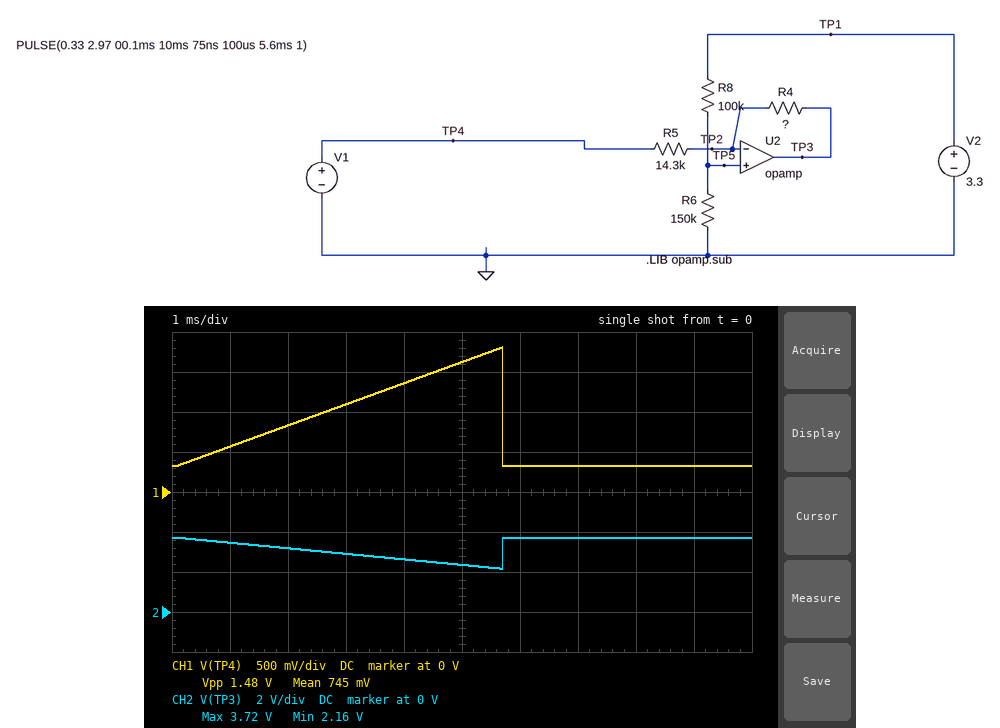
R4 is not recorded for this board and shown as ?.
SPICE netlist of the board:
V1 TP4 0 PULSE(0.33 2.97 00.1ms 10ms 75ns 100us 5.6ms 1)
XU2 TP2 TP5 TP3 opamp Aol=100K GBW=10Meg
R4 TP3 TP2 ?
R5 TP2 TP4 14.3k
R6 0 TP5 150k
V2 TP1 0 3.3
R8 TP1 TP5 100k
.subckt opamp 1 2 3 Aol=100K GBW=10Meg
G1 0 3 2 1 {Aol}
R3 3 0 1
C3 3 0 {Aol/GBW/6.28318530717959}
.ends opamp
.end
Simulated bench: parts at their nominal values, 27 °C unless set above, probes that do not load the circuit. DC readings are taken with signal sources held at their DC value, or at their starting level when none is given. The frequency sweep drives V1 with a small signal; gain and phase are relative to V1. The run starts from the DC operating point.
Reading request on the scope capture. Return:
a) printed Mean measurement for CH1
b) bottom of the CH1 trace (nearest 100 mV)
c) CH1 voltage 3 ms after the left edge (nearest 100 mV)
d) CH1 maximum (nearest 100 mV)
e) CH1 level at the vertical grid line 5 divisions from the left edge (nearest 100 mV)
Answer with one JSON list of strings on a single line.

["745 mV", "300 mV", "1.1 V", "1.8 V", "1.6 V"]
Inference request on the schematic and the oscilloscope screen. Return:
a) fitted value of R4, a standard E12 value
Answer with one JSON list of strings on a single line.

["15 kΩ"]
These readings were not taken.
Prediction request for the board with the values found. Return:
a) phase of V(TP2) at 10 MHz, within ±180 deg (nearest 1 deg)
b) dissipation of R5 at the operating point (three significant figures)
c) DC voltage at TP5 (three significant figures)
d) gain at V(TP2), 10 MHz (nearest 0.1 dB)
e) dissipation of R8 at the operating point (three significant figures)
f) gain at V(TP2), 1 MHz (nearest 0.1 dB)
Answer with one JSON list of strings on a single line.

["26 deg", "190 µW", "1.98 V", "-6.7 dB", "17.4 µW", "-19.8 dB"]
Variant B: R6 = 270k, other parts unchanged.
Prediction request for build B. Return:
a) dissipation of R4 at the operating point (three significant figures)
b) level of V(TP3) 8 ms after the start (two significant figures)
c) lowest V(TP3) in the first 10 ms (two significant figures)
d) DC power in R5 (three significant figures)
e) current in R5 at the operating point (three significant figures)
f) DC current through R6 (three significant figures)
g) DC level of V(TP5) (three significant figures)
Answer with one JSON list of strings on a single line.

["317 µW", "4.6 V", "3.0 V", "302 µW", "145 µA", "8.92 µA", "2.41 V"]
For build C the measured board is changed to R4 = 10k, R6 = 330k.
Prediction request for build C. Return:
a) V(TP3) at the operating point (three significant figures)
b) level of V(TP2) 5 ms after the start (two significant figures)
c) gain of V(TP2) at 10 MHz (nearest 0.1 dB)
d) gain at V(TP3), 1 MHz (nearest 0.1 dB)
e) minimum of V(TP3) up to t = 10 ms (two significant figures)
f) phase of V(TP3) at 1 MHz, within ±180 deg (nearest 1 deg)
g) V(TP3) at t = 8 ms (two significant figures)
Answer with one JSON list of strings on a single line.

["4.07 V", "2.5 V", "-9.0 dB", "-3.2 dB", "3.0 V", "170 deg", "4.1 V"]
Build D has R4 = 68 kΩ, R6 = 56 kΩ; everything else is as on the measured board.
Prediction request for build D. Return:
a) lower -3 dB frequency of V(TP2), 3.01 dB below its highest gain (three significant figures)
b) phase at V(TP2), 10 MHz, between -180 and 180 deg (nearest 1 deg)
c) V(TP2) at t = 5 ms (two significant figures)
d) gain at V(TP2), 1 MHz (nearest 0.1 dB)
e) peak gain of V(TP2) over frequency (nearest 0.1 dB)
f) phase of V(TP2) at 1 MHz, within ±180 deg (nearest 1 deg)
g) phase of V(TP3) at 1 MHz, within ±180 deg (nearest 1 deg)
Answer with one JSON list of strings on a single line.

["1.74 MHz", "10 deg", "1.2 V", "-7.7 dB", "-1.7 dB", "60 deg", "150 deg"]
